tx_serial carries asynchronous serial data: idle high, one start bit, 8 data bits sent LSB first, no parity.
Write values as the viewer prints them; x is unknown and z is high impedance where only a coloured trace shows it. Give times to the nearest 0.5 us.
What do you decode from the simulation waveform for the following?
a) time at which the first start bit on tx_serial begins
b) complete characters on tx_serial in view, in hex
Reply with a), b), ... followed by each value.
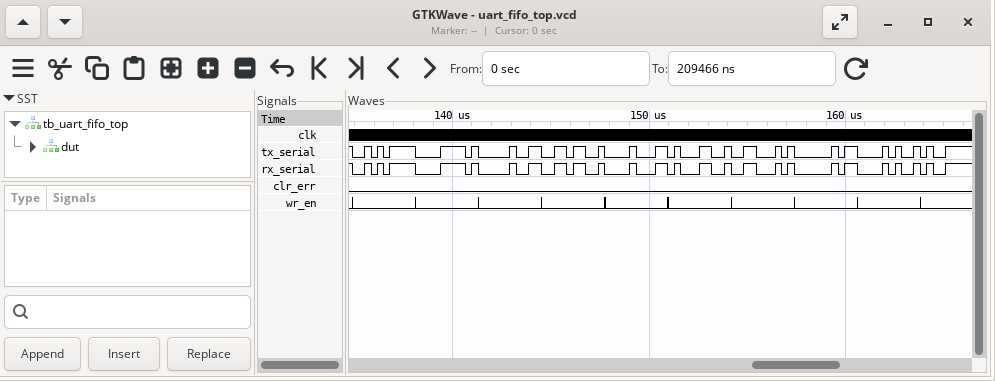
a) 135 us
b) EA, 78, 90, 36, 88, 31, 46, A0, 28
